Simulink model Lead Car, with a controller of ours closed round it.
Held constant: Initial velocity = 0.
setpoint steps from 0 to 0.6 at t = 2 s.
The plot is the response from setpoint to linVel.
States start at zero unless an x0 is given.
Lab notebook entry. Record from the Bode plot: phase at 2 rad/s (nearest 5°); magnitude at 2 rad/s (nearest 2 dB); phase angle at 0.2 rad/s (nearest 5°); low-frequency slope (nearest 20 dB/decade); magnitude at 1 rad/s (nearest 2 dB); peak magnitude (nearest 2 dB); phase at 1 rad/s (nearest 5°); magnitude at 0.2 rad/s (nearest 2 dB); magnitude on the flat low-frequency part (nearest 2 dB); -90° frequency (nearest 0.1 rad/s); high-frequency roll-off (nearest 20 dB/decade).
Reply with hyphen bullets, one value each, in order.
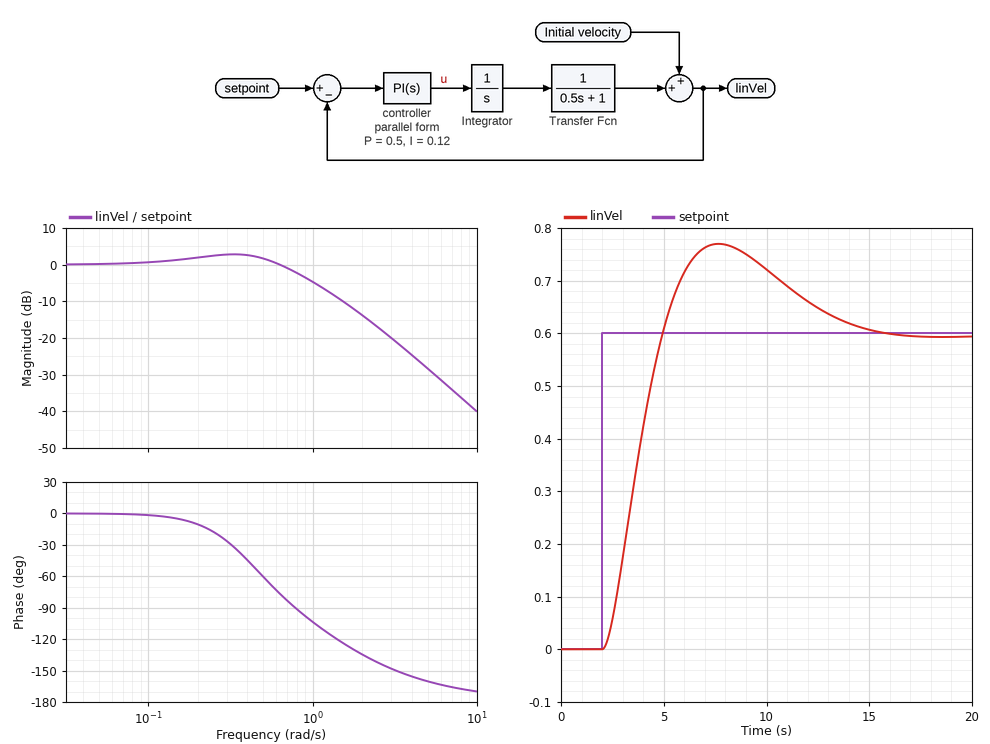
- -135°
- -14 dB
- -10°
- 0 dB/decade
- -4 dB
- 2 dB
- -105°
- 2 dB
- 0 dB
- 0.8 rad/s
- -40 dB/decade
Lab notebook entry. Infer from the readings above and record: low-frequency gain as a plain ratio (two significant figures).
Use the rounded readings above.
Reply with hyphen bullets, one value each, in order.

- 1.0
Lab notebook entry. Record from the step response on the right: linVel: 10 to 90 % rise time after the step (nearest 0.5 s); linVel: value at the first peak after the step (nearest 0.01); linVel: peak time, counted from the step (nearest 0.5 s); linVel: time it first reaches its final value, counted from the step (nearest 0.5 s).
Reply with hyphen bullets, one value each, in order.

- 2.0 s
- 0.77
- 5.5 s
- 3.0 s
